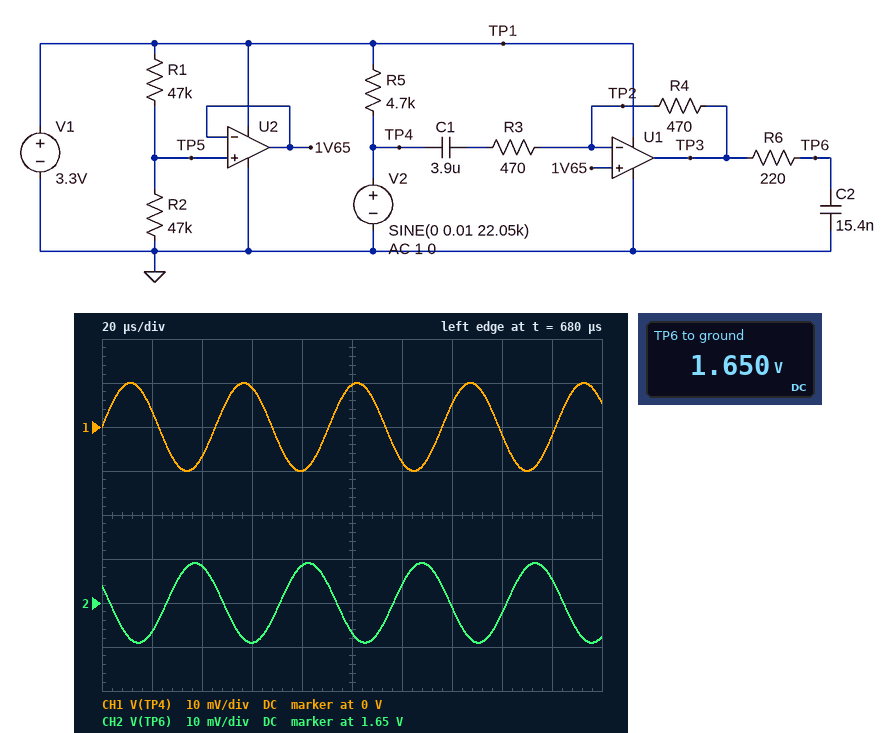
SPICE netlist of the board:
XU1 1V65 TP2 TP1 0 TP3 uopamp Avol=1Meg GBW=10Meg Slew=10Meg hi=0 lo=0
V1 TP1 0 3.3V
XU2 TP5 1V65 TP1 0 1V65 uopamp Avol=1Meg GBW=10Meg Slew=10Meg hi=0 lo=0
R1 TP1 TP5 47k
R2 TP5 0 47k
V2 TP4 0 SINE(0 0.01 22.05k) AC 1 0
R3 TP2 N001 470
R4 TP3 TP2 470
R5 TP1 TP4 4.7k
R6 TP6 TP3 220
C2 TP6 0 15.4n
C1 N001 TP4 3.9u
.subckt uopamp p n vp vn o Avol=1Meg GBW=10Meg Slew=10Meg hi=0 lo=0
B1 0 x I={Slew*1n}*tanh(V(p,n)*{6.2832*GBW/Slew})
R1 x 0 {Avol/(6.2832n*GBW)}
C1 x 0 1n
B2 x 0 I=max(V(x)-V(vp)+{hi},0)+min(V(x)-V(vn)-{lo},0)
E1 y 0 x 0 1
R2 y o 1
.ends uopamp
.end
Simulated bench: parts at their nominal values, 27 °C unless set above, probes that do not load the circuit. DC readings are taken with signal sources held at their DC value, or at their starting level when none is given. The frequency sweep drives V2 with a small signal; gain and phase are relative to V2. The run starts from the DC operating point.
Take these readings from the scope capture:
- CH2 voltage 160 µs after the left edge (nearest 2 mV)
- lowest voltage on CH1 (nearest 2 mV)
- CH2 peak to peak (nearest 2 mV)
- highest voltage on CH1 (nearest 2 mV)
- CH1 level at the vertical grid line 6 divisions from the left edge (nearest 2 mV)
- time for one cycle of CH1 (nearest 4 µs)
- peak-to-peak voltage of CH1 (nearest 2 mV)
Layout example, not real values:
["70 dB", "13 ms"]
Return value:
["1.648 V", "-10 mV", "18 mV", "10 mV", "-8 mV", "44 µs", "20 mV"]
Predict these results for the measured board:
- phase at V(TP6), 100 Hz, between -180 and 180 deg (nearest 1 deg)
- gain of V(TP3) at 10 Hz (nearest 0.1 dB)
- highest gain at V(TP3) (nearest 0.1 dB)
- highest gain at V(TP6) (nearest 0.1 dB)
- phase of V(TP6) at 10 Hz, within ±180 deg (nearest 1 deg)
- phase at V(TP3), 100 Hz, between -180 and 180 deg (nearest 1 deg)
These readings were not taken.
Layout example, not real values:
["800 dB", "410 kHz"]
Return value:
["-139 deg", "-18.8 dB", "0 dB", "0 dB", "-97 deg", "-139 deg"]
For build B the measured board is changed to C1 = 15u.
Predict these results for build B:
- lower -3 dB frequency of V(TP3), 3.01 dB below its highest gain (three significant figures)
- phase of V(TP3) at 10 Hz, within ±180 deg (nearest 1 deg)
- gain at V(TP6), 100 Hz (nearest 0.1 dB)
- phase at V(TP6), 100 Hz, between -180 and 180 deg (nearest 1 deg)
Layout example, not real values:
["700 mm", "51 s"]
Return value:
["22.6 Hz", "-114 deg", "-0.2 dB", "-167 deg"]
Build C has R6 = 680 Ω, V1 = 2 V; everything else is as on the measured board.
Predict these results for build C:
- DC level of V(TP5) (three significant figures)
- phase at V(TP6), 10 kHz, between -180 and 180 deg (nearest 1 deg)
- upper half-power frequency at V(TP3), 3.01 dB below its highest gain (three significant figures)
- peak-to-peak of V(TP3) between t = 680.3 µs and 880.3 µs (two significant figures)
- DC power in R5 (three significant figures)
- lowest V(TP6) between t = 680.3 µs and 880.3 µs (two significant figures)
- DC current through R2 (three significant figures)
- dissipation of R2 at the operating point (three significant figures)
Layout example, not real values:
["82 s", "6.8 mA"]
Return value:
["1.00 V", "147 deg", "4.99 MHz", "20 mV", "851 µW", "990 mV", "21.3 µA", "21.3 µW"]
